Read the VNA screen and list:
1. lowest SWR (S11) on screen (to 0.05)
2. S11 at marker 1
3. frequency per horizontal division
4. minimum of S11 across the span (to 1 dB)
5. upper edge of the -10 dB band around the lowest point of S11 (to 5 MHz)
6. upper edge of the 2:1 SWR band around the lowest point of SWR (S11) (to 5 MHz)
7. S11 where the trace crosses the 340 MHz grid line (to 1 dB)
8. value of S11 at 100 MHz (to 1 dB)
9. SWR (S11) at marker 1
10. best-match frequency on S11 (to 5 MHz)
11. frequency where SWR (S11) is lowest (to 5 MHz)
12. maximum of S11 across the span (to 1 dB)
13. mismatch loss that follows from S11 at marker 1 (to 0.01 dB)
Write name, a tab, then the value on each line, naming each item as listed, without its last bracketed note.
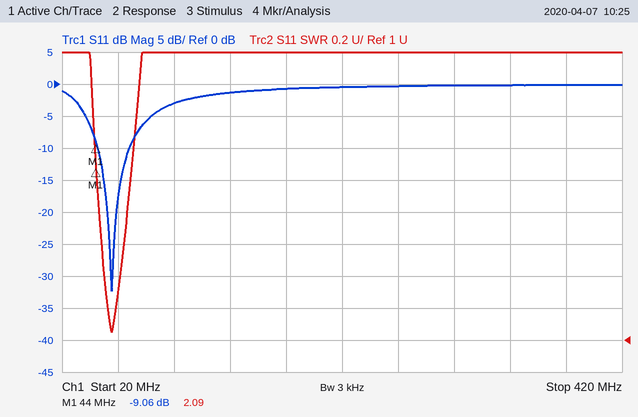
lowest SWR (S11) on screen	1.05
S11 at marker 1	-9.06 dB
frequency per horizontal division	40 MHz
minimum of S11 across the span	-32 dB
upper edge of the -10 dB band around the lowest point of S11	70 MHz
upper edge of the 2:1 SWR band around the lowest point of SWR (S11)	70 MHz
S11 where the trace crosses the 340 MHz grid line	0 dB
value of S11 at 100 MHz	-3 dB
SWR (S11) at marker 1	2.09
best-match frequency on S11	55 MHz
frequency where SWR (S11) is lowest	55 MHz
maximum of S11 across the span	0 dB
mismatch loss that follows from S11 at marker 1	0.58 dB
